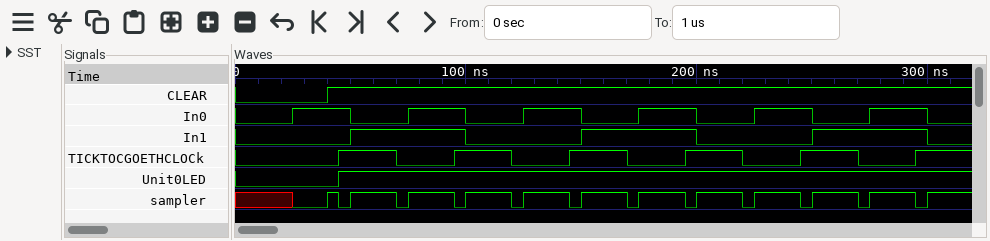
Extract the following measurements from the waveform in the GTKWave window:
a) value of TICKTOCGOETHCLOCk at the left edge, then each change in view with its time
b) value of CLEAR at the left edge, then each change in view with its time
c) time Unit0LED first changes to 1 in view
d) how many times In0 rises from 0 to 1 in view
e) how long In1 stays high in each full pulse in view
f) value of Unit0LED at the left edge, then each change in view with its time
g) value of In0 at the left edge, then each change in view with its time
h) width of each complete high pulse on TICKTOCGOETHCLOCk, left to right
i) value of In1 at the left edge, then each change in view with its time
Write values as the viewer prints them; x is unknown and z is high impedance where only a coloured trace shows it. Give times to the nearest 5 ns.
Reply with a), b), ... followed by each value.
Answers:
a) 0, 1 at 45 ns, 0 at 70 ns, 1 at 95 ns, 0 at 120 ns, 1 at 145 ns, 0 at 170 ns, 1 at 195 ns, 0 at 220 ns, 1 at 245 ns, 0 at 270 ns, 1 at 295 ns
b) 0, 1 at 40 ns
c) 45 ns
d) 6
e) 50 ns, 50 ns, 50 ns
f) 0, 1 at 45 ns
g) 0, 1 at 25 ns, 0 at 50 ns, 1 at 75 ns, 0 at 100 ns, 1 at 125 ns, 0 at 150 ns, 1 at 175 ns, 0 at 200 ns, 1 at 225 ns, 0 at 250 ns, 1 at 275 ns, 0 at 300 ns
h) 25 ns, 25 ns, 25 ns, 25 ns, 25 ns
i) 0, 1 at 50 ns, 0 at 100 ns, 1 at 150 ns, 0 at 200 ns, 1 at 250 ns, 0 at 300 ns
